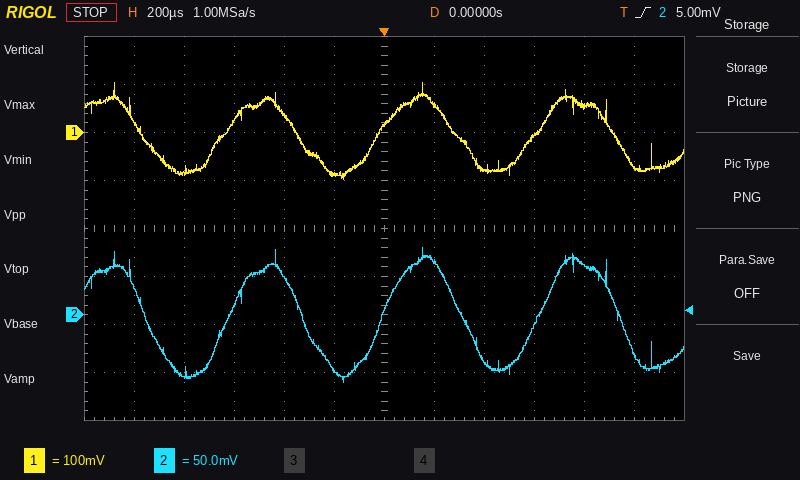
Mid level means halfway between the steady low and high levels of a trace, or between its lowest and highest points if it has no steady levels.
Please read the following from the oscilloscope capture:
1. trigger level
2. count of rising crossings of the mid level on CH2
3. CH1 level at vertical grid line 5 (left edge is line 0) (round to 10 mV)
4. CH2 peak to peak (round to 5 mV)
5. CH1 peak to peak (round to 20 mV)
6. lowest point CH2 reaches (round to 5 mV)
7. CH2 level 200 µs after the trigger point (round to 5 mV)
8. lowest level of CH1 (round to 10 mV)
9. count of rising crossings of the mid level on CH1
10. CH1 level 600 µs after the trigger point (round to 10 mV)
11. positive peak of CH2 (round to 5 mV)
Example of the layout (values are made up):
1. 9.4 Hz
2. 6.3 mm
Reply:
1. 5.00 mV
2. 3
3. -90 mV
4. 140 mV
5. 200 mV
6. -70 mV
7. 55 mV
8. -100 mV
9. 3
10. -10 mV
11. 70 mV
